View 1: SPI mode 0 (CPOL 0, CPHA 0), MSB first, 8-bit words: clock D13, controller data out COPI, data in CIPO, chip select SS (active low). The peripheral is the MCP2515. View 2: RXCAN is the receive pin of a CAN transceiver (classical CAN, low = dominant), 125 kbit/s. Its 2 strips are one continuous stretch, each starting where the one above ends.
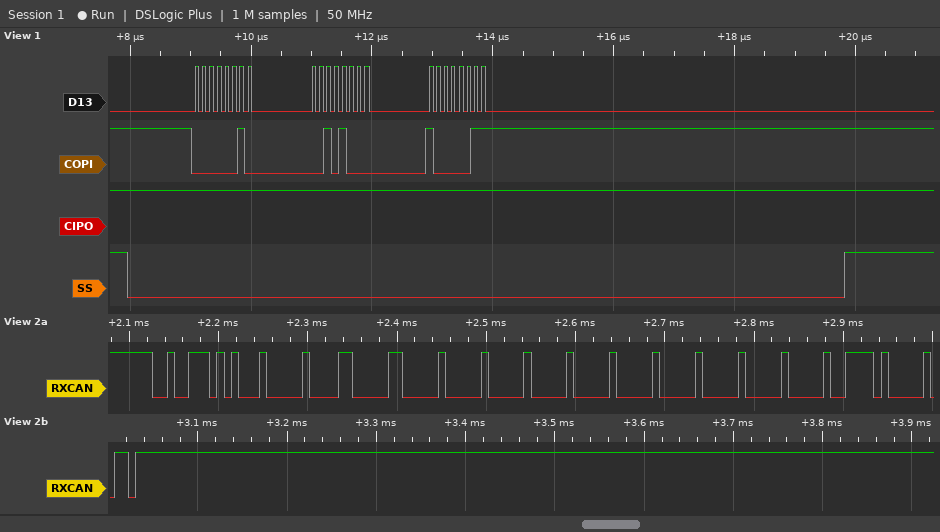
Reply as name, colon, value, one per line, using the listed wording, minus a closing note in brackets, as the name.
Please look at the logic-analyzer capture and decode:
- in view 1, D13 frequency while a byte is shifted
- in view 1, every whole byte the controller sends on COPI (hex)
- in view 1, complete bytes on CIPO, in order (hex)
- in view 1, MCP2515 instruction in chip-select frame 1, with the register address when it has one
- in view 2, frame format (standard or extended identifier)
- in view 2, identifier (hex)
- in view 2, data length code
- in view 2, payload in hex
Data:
in view 1, D13 frequency while a byte is shifted: 8 MHz
in view 1, every whole byte the controller sends on COPI: 02 28 83
in view 1, complete bytes on CIPO, in order: FF FF FF
in view 1, MCP2515 instruction in chip-select frame 1, with the register address when it has one: WRITE 0x28
in view 2, frame format: standard
in view 2, identifier: 0x275
in view 2, data length code: 8
in view 2, payload in hex: 03 04 00 00 00 00 00 00
